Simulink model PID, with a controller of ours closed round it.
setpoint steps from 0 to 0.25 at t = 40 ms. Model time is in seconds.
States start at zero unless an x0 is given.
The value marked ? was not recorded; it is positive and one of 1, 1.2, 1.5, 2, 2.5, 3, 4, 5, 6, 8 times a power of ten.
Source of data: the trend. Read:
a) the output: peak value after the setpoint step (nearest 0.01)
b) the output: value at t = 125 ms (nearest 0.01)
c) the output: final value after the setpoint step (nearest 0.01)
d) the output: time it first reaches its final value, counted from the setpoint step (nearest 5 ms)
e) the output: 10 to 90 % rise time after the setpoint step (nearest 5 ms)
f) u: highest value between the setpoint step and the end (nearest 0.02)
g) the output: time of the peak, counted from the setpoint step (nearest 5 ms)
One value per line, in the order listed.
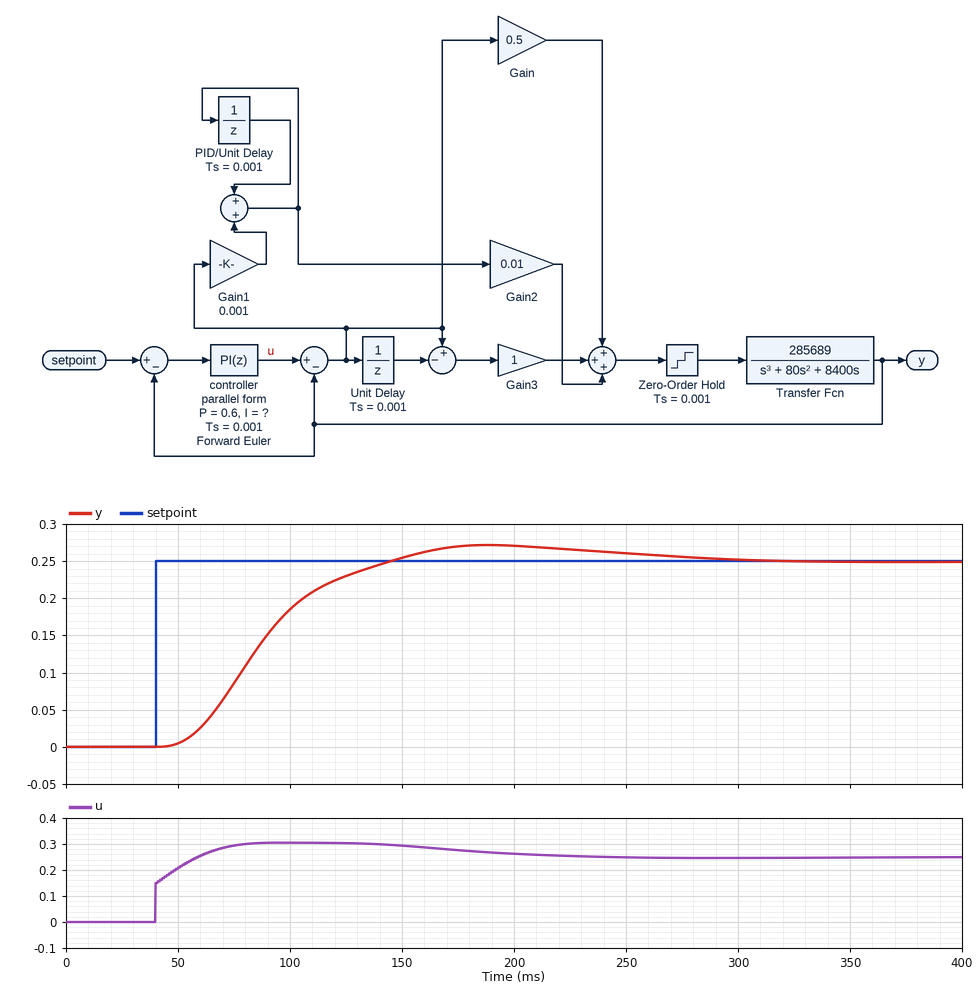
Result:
0.27
0.23
0.25
105 ms
60 ms
0.30
150 ms
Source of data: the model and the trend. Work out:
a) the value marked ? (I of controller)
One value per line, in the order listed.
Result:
25
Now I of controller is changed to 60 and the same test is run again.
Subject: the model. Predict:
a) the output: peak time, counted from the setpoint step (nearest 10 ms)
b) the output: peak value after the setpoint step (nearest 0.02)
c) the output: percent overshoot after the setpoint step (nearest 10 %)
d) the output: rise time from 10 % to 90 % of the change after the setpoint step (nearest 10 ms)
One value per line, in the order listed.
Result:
80 ms
0.36
50 %
30 ms
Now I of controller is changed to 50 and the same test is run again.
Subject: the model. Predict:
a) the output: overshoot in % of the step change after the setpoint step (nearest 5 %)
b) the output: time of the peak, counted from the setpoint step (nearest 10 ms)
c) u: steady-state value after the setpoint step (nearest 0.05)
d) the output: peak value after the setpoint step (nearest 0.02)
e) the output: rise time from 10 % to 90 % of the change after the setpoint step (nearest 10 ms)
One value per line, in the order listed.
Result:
35 %
90 ms
0.25
0.34
30 ms
